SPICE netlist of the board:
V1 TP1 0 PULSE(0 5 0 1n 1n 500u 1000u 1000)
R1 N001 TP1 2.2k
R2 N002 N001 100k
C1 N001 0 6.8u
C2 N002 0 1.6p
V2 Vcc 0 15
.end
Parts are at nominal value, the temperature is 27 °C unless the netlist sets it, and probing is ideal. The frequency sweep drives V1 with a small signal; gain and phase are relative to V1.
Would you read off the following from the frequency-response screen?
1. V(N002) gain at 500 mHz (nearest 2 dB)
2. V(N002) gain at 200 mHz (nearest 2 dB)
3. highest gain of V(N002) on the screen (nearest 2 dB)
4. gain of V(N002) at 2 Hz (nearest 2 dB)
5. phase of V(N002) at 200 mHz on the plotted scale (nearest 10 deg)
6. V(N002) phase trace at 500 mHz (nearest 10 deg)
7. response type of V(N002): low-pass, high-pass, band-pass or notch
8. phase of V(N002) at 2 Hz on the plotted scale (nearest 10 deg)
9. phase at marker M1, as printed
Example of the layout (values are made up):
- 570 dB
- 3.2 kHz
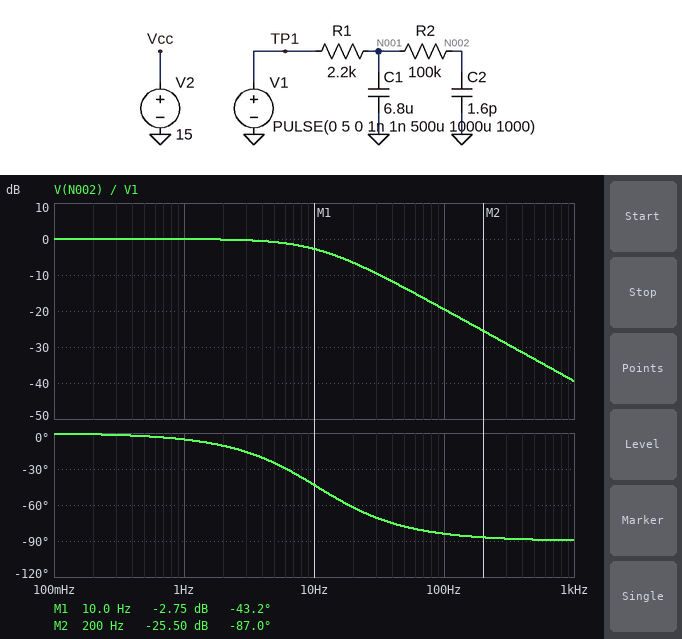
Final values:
- 0 dB
- 0 dB
- 0 dB
- 0 dB
- 0 deg
- 0 deg
- low-pass
- -10 deg
- -43.2 deg
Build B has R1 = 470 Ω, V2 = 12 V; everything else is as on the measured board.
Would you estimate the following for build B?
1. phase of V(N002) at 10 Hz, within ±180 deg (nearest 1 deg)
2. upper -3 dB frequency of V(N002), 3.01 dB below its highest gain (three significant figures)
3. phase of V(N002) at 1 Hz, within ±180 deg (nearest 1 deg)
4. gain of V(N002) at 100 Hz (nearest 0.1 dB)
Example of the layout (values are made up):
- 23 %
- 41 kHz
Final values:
- -11 deg
- 49.8 Hz
- -1 deg
- -7.0 dB
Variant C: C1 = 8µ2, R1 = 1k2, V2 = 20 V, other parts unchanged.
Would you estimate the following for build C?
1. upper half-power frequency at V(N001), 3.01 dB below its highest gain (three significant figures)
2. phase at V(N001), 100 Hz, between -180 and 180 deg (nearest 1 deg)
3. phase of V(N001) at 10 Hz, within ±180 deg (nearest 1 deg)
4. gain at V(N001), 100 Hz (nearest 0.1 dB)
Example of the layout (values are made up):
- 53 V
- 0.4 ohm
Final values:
- 16.2 Hz
- -81 deg
- -32 deg
- -15.9 dB
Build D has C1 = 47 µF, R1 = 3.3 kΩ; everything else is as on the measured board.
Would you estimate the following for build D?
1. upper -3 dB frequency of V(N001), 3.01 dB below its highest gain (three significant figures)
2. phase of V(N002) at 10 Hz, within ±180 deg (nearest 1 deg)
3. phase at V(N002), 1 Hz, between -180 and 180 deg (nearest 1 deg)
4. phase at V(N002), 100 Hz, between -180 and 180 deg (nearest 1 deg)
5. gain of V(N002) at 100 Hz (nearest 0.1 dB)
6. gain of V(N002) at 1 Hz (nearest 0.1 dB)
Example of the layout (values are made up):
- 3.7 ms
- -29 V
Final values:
- 1.03 Hz
- -84 deg
- -44 deg
- -89 deg
- -39.8 dB
- -2.9 dB
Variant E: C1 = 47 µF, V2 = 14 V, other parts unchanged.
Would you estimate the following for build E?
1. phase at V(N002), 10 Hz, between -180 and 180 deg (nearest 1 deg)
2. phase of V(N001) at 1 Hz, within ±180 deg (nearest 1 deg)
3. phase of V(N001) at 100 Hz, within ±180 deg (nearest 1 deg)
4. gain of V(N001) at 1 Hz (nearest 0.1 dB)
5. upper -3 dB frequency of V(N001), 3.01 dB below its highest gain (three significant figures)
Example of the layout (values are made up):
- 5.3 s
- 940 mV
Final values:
- -81 deg
- -33 deg
- -89 deg
- -1.5 dB
- 1.54 Hz
